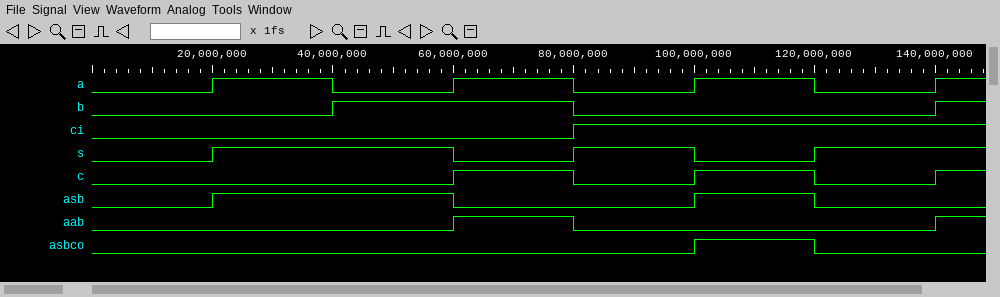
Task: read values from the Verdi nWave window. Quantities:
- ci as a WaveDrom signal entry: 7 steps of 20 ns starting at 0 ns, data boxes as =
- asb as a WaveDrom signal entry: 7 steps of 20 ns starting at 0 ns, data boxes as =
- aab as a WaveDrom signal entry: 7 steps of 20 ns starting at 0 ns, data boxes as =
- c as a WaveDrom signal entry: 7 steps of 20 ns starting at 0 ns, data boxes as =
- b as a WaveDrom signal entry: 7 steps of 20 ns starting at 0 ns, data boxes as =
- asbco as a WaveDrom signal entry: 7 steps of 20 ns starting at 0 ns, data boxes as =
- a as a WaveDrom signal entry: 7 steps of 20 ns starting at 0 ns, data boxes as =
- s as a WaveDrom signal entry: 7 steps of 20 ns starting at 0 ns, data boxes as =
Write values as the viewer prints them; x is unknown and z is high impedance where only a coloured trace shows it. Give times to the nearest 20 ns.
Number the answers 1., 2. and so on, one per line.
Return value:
1. {name: 'ci', wave: '0...1..'}
2. {name: 'asb', wave: '01.0.10'}
3. {name: 'aab', wave: '0..10..'}
4. {name: 'c', wave: '0..1010'}
5. {name: 'b', wave: '0.1.0..'}
6. {name: 'asbco', wave: '0....10'}
7. {name: 'a', wave: '0101010'}
8. {name: 's', wave: '01.0101'}
